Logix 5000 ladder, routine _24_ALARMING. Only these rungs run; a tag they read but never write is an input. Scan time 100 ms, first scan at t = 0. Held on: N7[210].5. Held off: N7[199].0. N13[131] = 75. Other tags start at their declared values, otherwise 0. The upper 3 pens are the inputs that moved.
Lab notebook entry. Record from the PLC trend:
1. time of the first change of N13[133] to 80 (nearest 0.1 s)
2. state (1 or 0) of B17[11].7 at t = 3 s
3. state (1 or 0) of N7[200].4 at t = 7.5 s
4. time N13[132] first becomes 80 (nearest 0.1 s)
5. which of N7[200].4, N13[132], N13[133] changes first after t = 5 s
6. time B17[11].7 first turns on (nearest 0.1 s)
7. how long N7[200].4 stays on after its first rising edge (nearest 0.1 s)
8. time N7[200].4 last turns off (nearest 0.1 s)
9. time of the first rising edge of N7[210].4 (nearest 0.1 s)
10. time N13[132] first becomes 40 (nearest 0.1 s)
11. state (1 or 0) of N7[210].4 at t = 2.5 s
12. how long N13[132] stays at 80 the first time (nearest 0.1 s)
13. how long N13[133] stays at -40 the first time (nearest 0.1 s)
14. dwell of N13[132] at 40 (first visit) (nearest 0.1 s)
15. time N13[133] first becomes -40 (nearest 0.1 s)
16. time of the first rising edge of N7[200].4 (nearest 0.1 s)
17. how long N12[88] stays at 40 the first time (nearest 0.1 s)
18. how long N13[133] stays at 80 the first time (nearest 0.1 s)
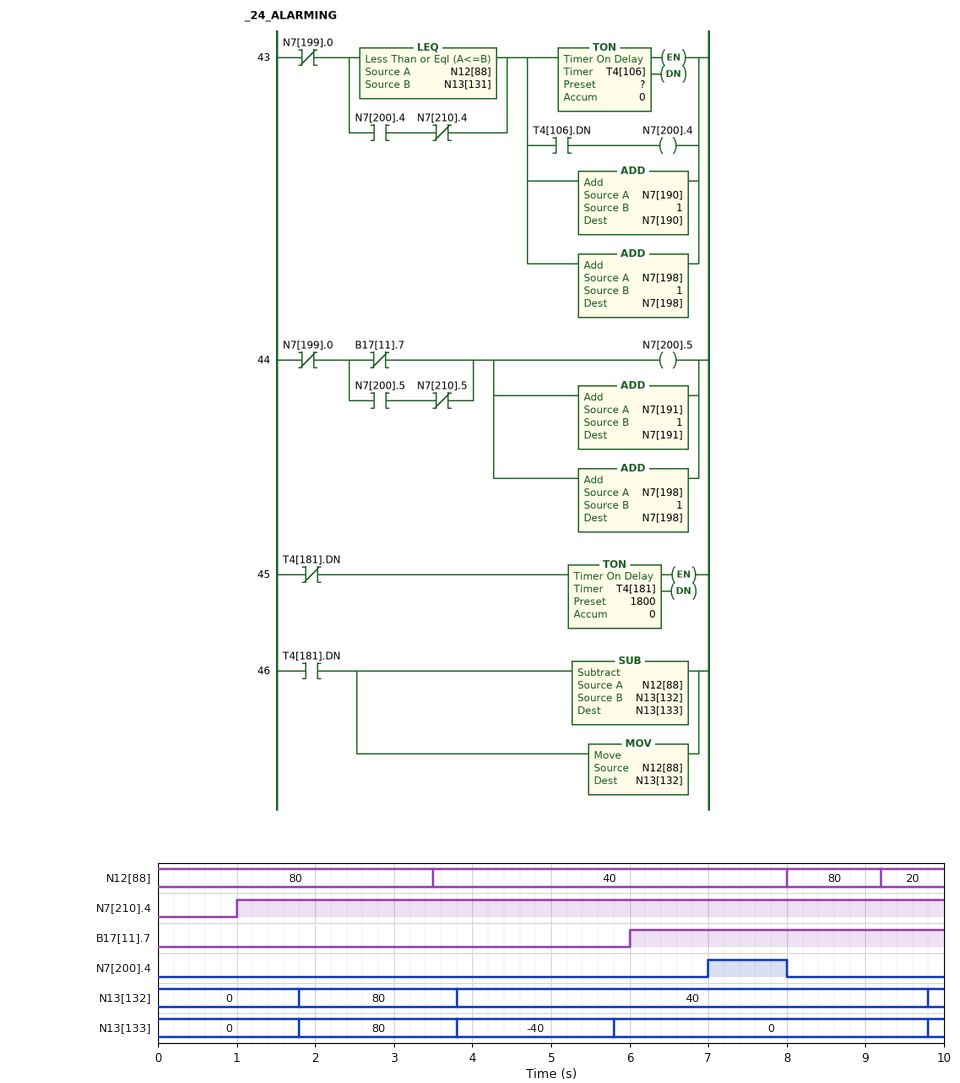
1.8 s
0
1
1.8 s
N13[133]
6.0 s
1.0 s
8.0 s
1.0 s
3.8 s
1
2.0 s
2.0 s
6.0 s
3.8 s
7.0 s
4.5 s
2.0 s
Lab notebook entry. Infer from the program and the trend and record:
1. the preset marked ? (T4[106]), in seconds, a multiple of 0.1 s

3.5 s
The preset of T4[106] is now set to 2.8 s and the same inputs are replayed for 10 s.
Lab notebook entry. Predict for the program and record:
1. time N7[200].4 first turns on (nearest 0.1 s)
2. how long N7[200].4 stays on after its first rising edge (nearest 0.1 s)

6.3 s
1.7 s
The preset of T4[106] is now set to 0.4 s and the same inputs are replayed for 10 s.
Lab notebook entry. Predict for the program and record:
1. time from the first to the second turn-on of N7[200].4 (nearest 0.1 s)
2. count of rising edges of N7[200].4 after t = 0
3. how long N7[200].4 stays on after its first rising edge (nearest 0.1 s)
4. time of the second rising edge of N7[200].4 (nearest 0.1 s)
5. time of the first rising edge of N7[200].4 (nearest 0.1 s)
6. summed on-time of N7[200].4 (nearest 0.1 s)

5.7 s
2
4.1 s
9.6 s
3.9 s
4.5 s
